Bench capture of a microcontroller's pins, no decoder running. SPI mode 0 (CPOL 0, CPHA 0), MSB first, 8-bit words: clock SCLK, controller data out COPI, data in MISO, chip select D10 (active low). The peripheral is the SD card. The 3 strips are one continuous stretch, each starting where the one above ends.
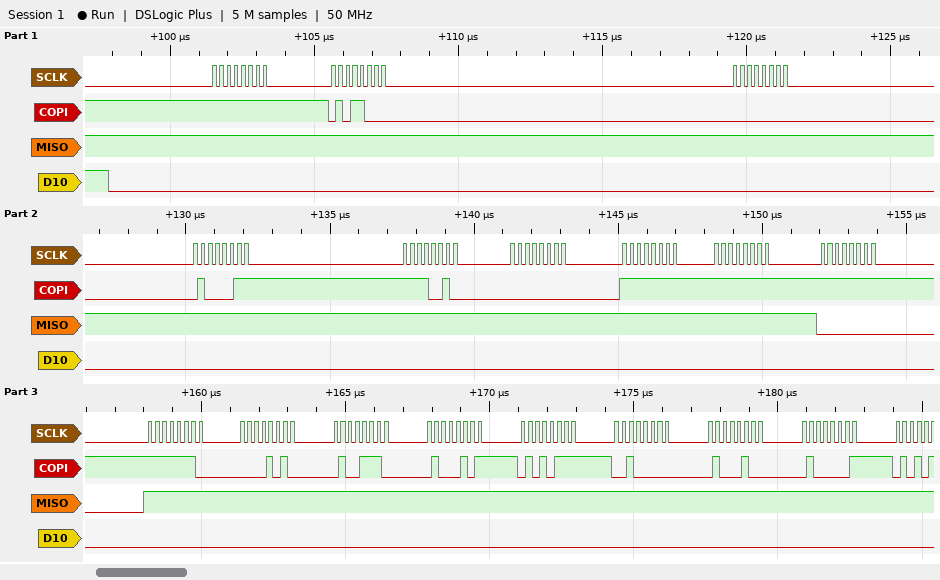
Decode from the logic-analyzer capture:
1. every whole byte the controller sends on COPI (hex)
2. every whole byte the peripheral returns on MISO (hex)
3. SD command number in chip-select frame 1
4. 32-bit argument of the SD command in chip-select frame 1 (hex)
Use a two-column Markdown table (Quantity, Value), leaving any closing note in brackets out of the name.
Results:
| Quantity | Value |
|---|---|
| every whole byte the controller sends on COPI | FF 58 00 43 F2 00 FF FF FF FE 0A 4E 45 57 20 44 41 |
| every whole byte the peripheral returns on MISO | FF FF FF FF FF FF FF FF 00 FF FF FF FF FF FF FF FF |
| SD command number in chip-select frame 1 | CMD24 |
| 32-bit argument of the SD command in chip-select frame 1 | 0x0043F200 |
